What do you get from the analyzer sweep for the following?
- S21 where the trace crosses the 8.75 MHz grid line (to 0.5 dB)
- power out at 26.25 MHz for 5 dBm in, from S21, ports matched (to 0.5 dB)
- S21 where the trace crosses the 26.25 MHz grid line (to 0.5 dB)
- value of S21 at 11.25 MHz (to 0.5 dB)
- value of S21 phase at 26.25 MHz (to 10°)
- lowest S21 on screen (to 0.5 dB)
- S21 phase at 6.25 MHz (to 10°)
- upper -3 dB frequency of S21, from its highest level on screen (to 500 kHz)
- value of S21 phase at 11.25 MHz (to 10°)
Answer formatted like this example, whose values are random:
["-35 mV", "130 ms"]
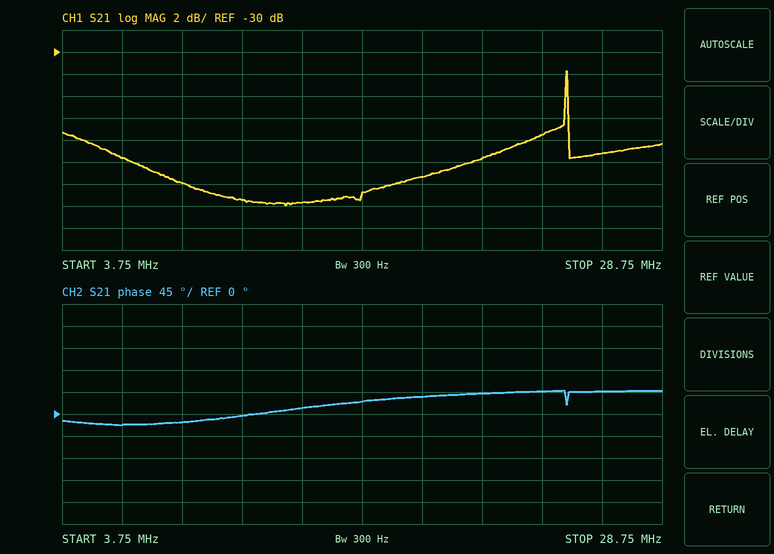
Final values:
["-42.0 dB", "-34.0 dBm", "-39.0 dB", "-43.5 dB", "50°", "-44.0 dB", "-20°", "25.0 MHz", "0°"]
